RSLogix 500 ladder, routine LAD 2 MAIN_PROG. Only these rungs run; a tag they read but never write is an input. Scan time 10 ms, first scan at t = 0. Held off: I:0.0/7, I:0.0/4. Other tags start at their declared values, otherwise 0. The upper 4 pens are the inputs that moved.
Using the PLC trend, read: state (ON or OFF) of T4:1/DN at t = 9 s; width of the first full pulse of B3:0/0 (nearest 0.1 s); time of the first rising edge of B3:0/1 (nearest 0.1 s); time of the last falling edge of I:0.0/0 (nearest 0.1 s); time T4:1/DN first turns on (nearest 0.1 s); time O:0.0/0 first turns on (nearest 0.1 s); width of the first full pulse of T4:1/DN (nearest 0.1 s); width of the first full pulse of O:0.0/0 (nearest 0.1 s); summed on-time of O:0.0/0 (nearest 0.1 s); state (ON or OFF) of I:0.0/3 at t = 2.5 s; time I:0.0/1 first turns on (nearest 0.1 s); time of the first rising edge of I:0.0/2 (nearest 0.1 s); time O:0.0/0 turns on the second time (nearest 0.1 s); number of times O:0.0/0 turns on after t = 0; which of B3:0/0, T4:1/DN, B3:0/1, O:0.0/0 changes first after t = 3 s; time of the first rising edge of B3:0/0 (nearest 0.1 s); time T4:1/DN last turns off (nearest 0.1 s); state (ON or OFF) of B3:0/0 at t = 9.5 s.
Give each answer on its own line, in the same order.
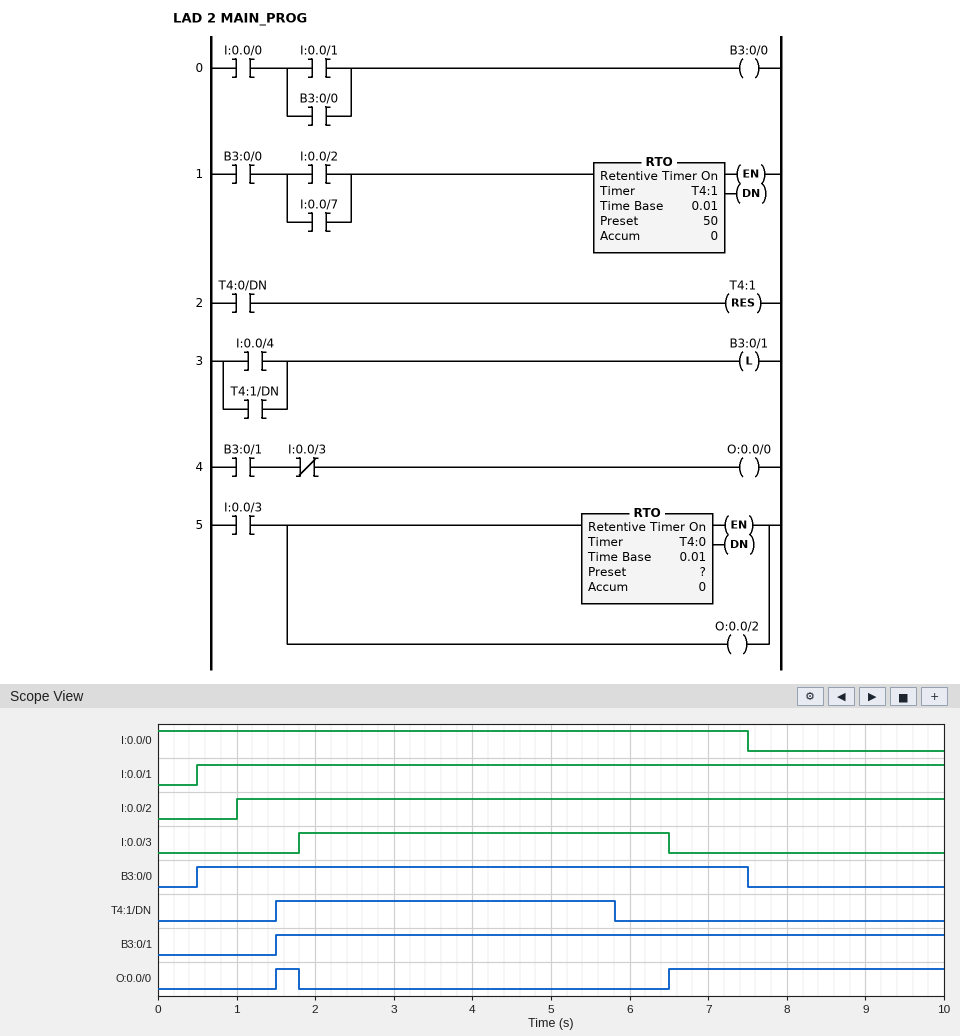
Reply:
OFF
7.0 s
1.5 s
7.5 s
1.5 s
1.5 s
4.3 s
0.3 s
3.8 s
ON
0.5 s
1.0 s
6.5 s
2
T4:1/DN
0.5 s
5.8 s
OFF
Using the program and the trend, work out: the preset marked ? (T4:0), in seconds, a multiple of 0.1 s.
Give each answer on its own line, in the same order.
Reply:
4.0 s
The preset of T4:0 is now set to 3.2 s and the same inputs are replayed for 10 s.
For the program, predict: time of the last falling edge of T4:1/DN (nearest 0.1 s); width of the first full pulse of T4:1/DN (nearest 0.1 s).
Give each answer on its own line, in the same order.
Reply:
5.0 s
3.5 s
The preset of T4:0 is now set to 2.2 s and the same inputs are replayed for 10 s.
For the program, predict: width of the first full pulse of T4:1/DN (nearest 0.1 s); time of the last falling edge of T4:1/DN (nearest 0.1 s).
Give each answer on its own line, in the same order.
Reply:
2.5 s
4.0 s
